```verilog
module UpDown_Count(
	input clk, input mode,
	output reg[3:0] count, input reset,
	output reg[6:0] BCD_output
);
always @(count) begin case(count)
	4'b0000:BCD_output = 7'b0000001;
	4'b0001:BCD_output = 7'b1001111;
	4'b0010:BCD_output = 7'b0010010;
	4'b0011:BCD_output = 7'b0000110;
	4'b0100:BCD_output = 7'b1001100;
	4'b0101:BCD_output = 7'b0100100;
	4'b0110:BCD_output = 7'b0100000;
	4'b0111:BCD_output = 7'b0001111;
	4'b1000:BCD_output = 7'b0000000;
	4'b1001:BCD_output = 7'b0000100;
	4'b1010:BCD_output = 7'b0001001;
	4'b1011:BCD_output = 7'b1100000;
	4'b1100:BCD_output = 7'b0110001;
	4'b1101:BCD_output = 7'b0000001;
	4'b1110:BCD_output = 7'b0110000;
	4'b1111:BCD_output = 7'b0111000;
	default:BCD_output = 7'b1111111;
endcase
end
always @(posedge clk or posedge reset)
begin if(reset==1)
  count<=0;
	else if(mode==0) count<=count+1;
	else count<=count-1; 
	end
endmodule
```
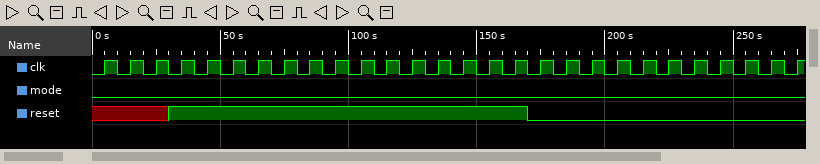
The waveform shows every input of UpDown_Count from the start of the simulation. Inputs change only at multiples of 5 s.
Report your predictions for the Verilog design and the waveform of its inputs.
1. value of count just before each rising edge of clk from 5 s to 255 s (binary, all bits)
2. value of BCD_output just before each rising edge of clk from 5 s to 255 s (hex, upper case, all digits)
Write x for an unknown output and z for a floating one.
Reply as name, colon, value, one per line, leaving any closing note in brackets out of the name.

value of count just before each rising edge of clk from 5 s to 255 s: x, x, x, 0000, 0000, 0000, 0000, 0000, 0000, 0000, 0000, 0000, 0000, 0000, 0000, 0000, 0000, 0000, 0001, 0010, 0011, 0100, 0101, 0110, 0111, 1000
value of BCD_output just before each rising edge of clk from 5 s to 255 s: x, x, x, 01, 01, 01, 01, 01, 01, 01, 01, 01, 01, 01, 01, 01, 01, 01, 4F, 12, 06, 4C, 24, 20, 0F, 00
